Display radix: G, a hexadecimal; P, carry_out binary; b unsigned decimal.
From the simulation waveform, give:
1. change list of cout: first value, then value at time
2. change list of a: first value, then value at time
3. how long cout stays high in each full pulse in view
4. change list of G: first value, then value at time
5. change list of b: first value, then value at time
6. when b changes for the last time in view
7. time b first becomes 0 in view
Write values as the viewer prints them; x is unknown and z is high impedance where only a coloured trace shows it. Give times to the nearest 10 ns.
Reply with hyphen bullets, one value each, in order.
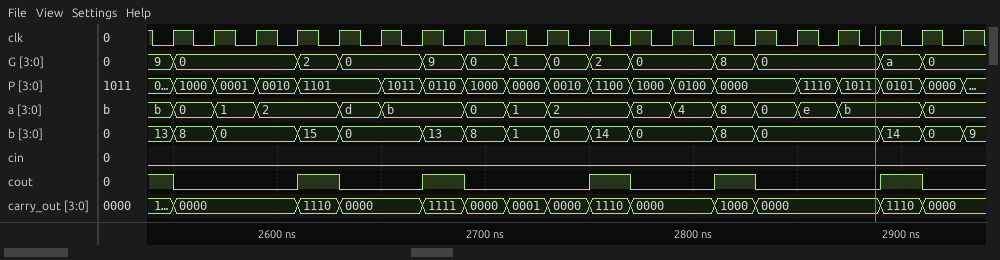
- 1, 0 at 2550 ns, 1 at 2610 ns, 0 at 2630 ns, 1 at 2670 ns, 0 at 2690 ns, 1 at 2750 ns, 0 at 2770 ns, 1 at 2810 ns, 0 at 2830 ns, 1 at 2890 ns, 0 at 2910 ns
- b, 0 at 2550 ns, 1 at 2570 ns, 2 at 2590 ns, d at 2630 ns, b at 2650 ns, 0 at 2690 ns, 1 at 2710 ns, 2 at 2730 ns, 8 at 2770 ns, 4 at 2790 ns, 8 at 2810 ns, 0 at 2830 ns, e at 2850 ns, b at 2870 ns, 0 at 2910 ns
- 20 ns, 20 ns, 20 ns, 20 ns, 20 ns
- 9, 0 at 2550 ns, 2 at 2610 ns, 0 at 2630 ns, 9 at 2670 ns, 0 at 2690 ns, 1 at 2710 ns, 0 at 2730 ns, 2 at 2750 ns, 0 at 2770 ns, 8 at 2810 ns, 0 at 2830 ns, a at 2890 ns, 0 at 2910 ns
- 13, 8 at 2550 ns, 0 at 2570 ns, 15 at 2610 ns, 0 at 2630 ns, 13 at 2670 ns, 8 at 2690 ns, 1 at 2710 ns, 0 at 2730 ns, 14 at 2750 ns, 0 at 2770 ns, 8 at 2810 ns, 0 at 2830 ns, 14 at 2890 ns, 0 at 2910 ns, 9 at 2930 ns
- 2930 ns
- 2570 ns
